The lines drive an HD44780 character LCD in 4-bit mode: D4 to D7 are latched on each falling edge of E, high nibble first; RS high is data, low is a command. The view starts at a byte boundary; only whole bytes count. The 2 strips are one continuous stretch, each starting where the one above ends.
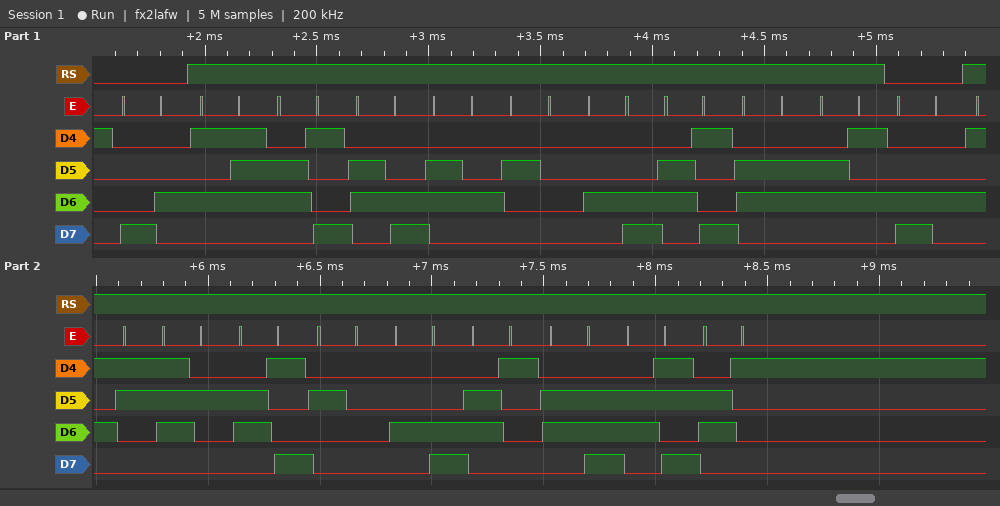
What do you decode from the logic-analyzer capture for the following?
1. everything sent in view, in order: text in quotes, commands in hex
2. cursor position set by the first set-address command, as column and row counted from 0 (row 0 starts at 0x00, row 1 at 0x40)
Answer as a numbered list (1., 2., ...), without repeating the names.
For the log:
1. 0x84 "Wild Life" 0xC4 "Sri Lanka"
2. column 4, row 0
